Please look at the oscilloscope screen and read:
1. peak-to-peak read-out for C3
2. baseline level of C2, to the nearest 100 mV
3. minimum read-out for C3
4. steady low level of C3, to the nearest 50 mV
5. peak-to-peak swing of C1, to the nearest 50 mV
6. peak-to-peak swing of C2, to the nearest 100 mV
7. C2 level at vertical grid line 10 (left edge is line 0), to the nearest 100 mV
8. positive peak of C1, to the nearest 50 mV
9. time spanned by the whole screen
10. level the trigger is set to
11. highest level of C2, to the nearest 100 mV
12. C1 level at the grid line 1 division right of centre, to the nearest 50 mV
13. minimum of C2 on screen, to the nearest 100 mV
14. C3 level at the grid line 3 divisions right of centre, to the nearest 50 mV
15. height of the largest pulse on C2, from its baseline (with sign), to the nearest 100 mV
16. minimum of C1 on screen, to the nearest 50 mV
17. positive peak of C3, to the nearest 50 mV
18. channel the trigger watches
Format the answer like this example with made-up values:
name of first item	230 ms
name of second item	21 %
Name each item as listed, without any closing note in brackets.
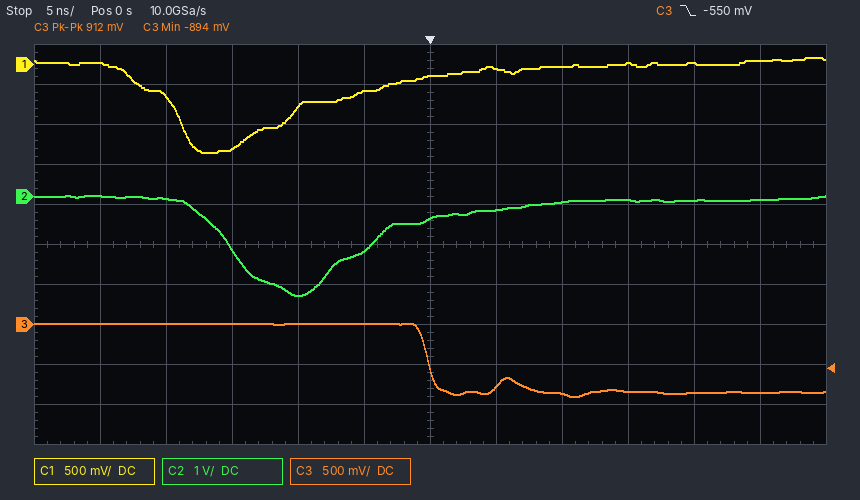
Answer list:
peak-to-peak read-out for C3	912 mV
baseline level of C2, to the nearest 100 mV	-100 mV
minimum read-out for C3	-894 mV
steady low level of C3, to the nearest 50 mV	-850 mV
peak-to-peak swing of C1, to the nearest 50 mV	1.20 V
peak-to-peak swing of C2, to the nearest 100 mV	2.5 V
C2 level at vertical grid line 10 (left edge is line 0), to the nearest 100 mV	-100 mV
positive peak of C1, to the nearest 50 mV	100 mV
time spanned by the whole screen	60 ns
level the trigger is set to	-550 mV
highest level of C2, to the nearest 100 mV	0.0 V
C1 level at the grid line 1 division right of centre, to the nearest 50 mV	-50 mV
minimum of C2 on screen, to the nearest 100 mV	-2.5 V
C3 level at the grid line 3 divisions right of centre, to the nearest 50 mV	-850 mV
height of the largest pulse on C2, from its baseline (with sign), to the nearest 100 mV	-2.4 V
minimum of C1 on screen, to the nearest 50 mV	-1.10 V
positive peak of C3, to the nearest 50 mV	0 mV
channel the trigger watches	C3
